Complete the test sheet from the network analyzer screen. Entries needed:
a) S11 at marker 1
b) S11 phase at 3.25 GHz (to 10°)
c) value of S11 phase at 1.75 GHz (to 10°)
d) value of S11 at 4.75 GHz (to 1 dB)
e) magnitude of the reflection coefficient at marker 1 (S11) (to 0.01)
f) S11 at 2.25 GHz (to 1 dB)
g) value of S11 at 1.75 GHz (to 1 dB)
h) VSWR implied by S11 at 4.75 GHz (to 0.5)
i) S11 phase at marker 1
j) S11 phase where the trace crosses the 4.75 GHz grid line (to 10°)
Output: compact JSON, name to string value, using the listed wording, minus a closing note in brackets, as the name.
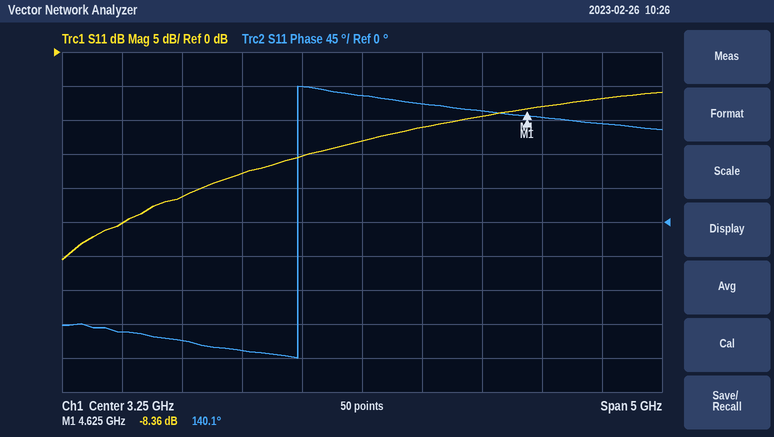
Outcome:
{"S11 at marker 1": "-8.36 dB", "S11 phase at 3.25 GHz": "170°", "value of S11 phase at 1.75 GHz": "-160°", "value of S11 at 4.75 GHz": "-8 dB", "magnitude of the reflection coefficient at marker 1 (S11)": "0.38", "S11 at 2.25 GHz": "-18 dB", "value of S11 at 1.75 GHz": "-21 dB", "VSWR implied by S11 at 4.75 GHz": "2.5", "S11 phase at marker 1": "140.1°", "S11 phase where the trace crosses the 4.75 GHz grid line": "140°"}
